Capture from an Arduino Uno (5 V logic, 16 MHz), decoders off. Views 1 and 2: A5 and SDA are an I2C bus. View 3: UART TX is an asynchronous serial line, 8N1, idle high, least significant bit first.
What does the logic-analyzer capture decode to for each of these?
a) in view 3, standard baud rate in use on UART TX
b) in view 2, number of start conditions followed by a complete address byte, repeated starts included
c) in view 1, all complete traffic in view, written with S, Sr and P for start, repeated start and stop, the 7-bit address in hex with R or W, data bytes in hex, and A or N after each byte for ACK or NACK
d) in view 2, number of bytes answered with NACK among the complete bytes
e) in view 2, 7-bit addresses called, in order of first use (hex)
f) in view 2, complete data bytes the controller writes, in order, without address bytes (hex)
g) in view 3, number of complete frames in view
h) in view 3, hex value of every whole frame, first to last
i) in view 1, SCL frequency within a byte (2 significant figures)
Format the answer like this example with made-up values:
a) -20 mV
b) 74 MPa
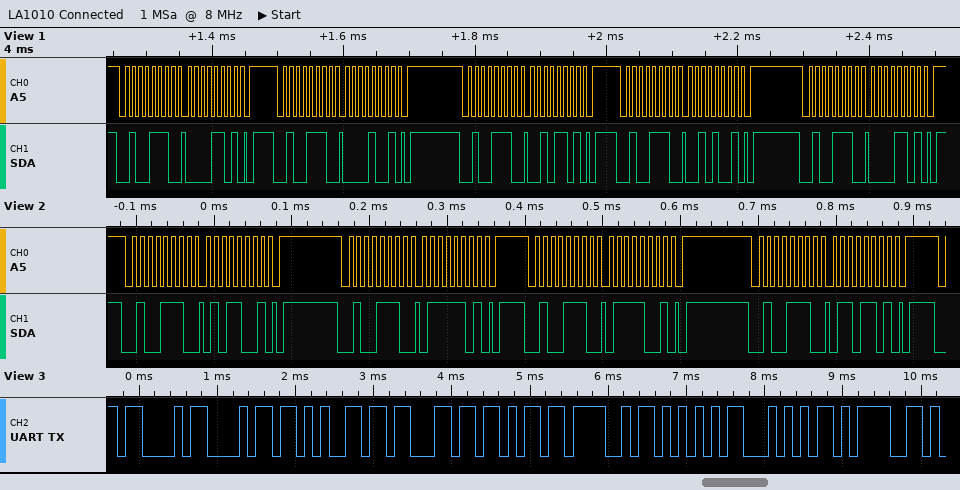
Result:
a) 9600 baud
b) 4
c) S 27W A 0D A P S 27W A 09 A P S 27W A 2D A P S 27W A 29 A P S 27W A 0D A P
d) 0
e) 0x27
f) 59 7D 79 6D
g) 9
h) 43 68 65 63 6B 4F 55 54 3D
i) 100 kHz
